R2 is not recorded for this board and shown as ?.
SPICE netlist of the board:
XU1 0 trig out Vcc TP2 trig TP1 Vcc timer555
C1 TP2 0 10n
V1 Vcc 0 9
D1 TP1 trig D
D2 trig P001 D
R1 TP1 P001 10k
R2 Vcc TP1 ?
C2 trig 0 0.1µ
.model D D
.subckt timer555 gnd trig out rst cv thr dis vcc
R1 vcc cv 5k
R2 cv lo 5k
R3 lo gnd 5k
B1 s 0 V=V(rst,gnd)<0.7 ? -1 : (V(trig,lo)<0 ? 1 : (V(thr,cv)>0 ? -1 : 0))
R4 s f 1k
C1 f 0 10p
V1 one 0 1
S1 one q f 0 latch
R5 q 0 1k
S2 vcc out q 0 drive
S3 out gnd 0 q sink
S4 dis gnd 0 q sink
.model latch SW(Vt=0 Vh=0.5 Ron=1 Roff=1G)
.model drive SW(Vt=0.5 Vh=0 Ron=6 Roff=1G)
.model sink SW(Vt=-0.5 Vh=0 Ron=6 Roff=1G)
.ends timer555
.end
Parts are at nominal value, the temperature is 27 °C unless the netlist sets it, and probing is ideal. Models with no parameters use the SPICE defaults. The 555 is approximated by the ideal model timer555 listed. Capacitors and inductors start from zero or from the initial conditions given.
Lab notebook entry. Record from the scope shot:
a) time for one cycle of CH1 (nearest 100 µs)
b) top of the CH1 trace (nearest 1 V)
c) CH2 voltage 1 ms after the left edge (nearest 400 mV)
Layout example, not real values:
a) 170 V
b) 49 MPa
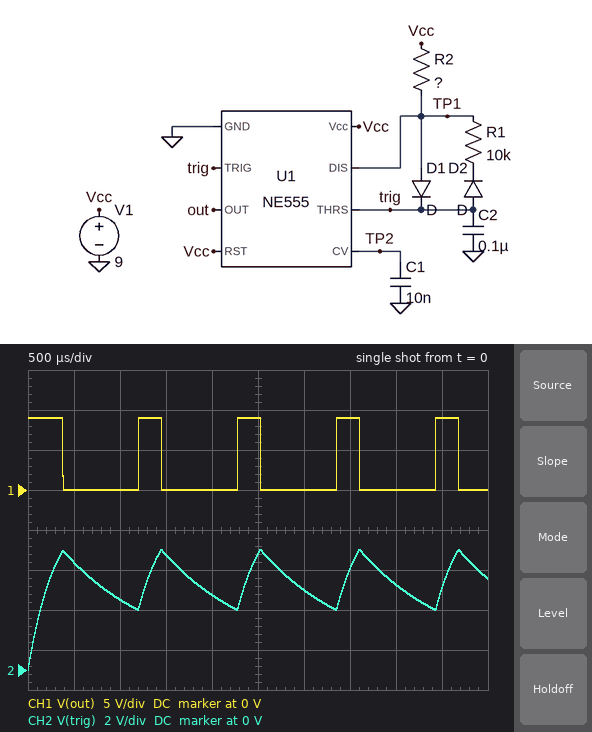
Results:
a) 1.1 ms
b) 9 V
c) 3.6 V
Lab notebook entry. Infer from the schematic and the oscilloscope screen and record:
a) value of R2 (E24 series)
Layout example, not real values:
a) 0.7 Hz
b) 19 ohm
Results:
a) 3 kΩ
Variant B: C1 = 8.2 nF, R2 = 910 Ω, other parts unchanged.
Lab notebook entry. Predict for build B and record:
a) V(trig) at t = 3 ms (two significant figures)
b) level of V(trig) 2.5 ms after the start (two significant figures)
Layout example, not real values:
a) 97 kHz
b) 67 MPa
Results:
a) 5.1 V
b) 3.6 V
